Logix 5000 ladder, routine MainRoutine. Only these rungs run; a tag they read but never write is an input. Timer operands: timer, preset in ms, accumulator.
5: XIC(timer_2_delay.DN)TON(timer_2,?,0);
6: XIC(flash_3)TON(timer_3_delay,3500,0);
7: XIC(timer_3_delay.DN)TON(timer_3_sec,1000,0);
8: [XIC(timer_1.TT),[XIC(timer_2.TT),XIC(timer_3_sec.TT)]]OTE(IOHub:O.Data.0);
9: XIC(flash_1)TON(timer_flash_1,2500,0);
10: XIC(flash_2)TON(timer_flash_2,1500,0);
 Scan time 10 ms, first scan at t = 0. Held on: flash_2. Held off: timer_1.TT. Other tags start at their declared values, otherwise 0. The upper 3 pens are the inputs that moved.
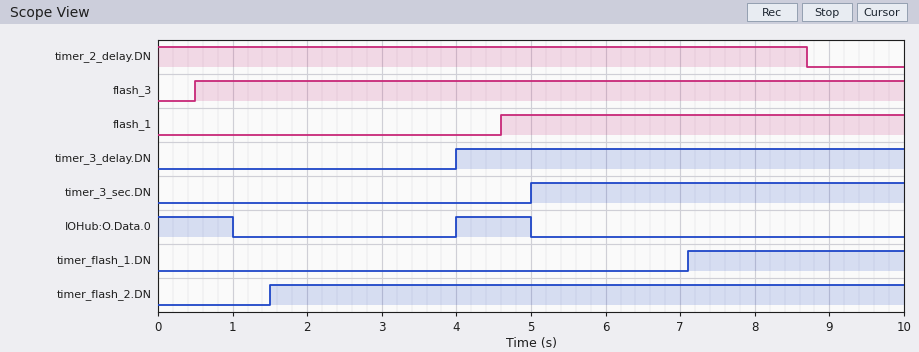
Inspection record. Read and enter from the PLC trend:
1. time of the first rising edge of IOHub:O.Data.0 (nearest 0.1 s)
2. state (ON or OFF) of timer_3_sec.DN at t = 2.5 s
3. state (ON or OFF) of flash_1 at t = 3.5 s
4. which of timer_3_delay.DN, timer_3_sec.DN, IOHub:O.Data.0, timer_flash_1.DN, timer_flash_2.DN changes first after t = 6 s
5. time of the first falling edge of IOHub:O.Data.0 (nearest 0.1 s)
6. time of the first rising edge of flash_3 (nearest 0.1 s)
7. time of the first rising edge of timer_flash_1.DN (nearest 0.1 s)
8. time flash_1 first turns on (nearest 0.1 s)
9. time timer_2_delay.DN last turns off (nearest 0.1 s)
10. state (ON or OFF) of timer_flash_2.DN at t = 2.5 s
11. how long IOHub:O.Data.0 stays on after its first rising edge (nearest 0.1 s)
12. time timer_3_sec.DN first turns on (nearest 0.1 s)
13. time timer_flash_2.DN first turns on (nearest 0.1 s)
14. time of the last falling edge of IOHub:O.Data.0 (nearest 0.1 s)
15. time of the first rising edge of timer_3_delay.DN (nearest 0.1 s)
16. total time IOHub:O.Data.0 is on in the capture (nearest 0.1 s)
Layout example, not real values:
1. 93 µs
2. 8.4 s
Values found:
1. 4.0 s
2. OFF
3. OFF
4. timer_flash_1.DN
5. 1.0 s
6. 0.5 s
7. 7.1 s
8. 4.6 s
9. 8.7 s
10. ON
11. 1.0 s
12. 5.0 s
13. 1.5 s
14. 5.0 s
15. 4.0 s
16. 2.0 s
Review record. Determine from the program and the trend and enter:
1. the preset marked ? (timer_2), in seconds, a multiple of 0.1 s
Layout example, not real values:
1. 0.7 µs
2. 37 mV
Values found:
1. 1.0 s
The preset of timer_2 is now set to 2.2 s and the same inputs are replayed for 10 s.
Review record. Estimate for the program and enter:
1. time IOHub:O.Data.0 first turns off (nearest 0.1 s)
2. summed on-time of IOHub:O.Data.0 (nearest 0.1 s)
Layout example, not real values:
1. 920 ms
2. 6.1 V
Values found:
1. 2.2 s
2. 3.2 s
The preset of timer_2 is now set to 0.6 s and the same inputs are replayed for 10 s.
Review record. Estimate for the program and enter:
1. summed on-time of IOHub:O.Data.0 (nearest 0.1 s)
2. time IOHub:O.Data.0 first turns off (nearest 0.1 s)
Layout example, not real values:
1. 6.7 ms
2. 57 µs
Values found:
1. 1.6 s
2. 0.6 s
